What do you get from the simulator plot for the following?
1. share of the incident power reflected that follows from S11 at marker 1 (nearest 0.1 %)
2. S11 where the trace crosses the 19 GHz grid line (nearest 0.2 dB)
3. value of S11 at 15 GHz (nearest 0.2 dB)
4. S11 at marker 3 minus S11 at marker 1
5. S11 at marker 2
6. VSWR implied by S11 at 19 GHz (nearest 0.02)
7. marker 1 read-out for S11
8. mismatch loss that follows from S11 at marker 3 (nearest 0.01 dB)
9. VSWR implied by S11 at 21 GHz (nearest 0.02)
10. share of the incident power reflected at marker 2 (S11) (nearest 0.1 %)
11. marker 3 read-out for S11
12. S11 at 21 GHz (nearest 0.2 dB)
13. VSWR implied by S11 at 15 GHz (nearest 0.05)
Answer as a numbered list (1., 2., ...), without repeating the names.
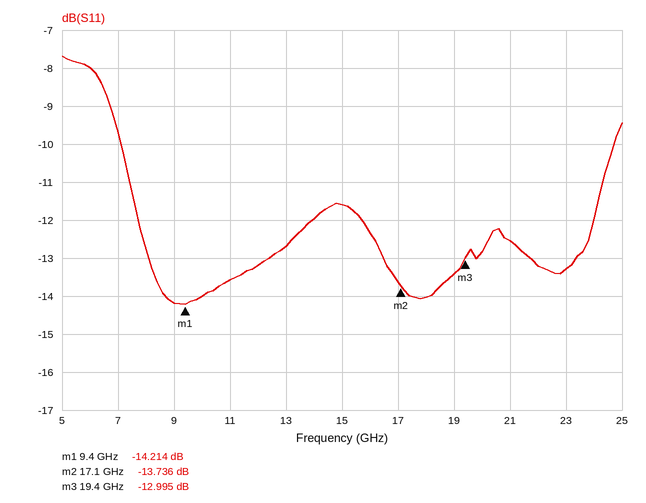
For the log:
1. 3.8 %
2. -13.4 dB
3. -11.6 dB
4. 1.219 dB
5. -13.736 dB
6. 1.54
7. -14.214 dB
8. 0.22 dB
9. 1.62
10. 4.2 %
11. -12.995 dB
12. -12.6 dB
13. 1.70
